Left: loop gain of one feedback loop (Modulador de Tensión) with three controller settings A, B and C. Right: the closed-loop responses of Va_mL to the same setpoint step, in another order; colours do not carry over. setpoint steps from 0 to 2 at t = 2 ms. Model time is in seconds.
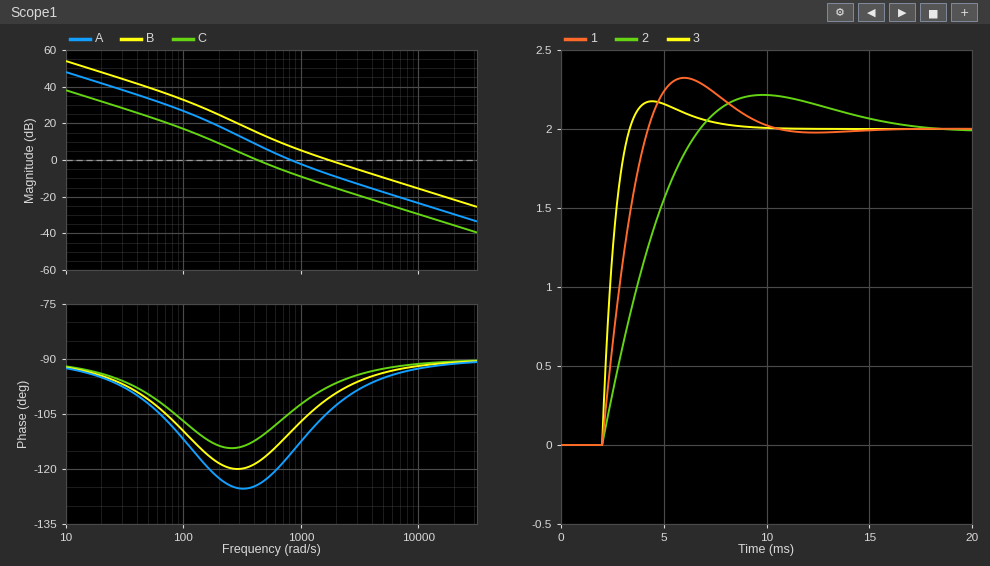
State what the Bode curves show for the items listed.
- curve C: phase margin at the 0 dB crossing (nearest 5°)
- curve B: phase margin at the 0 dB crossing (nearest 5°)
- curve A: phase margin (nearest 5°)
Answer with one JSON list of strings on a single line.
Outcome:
["70°", "80°", "65°"]
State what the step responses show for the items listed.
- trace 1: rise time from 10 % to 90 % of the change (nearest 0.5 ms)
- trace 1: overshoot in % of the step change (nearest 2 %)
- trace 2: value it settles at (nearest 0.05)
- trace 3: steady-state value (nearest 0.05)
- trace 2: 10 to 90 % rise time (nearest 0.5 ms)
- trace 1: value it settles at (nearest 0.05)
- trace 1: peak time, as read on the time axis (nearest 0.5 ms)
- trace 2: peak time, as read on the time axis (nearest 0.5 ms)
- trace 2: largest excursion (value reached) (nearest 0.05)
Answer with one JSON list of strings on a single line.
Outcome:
["1.5 ms", "16 %", "2.00", "2.00", "3.5 ms", "2.00", "6.0 ms", "10.0 ms", "2.20"]
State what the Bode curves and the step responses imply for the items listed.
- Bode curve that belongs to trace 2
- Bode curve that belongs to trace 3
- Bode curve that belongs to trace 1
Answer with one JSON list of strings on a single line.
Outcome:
["C", "B", "A"]
